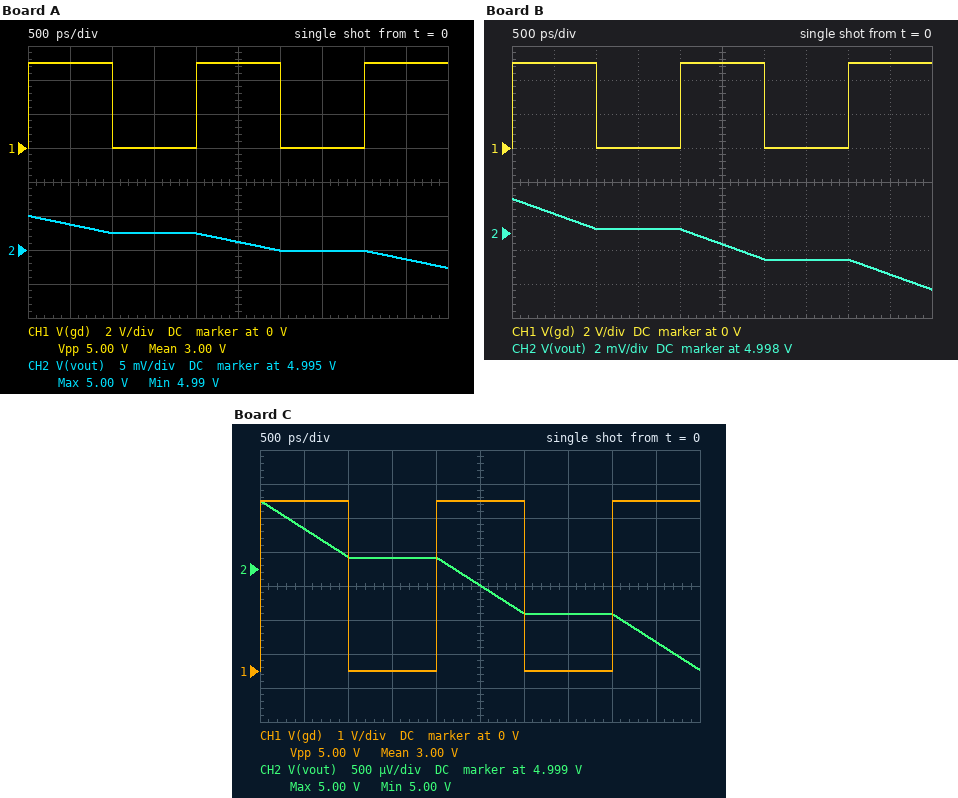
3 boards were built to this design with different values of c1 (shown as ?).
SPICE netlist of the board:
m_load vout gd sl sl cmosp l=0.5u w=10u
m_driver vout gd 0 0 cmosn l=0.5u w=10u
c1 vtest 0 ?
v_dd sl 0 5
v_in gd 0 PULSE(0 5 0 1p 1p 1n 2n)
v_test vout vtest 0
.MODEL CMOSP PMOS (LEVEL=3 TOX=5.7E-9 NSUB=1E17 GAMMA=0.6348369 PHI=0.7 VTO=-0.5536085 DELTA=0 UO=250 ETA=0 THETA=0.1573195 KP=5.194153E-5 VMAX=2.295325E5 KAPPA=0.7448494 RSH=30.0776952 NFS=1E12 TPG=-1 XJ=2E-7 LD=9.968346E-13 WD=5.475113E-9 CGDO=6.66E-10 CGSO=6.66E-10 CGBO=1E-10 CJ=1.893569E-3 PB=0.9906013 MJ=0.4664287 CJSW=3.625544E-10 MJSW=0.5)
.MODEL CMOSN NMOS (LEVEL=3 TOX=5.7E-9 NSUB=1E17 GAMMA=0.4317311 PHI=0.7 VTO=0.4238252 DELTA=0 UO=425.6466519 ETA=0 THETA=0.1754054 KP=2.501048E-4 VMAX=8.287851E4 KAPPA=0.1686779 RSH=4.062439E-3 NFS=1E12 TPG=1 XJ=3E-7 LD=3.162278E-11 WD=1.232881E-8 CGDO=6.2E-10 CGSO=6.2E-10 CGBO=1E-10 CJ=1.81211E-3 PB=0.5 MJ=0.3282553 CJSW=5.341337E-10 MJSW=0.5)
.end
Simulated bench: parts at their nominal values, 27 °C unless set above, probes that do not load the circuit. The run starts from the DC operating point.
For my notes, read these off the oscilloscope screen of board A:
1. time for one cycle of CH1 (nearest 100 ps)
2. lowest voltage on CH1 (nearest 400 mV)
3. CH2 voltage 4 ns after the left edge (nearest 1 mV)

2.0 ns
0 V
4.995 V
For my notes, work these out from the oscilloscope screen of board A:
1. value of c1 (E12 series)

3.9 nF
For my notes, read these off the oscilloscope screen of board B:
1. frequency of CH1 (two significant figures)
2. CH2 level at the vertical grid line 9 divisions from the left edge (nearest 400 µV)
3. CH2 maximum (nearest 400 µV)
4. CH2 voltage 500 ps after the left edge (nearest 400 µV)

500 MHz
4.9956 V
5.0000 V
4.9992 V
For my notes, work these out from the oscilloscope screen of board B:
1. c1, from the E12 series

5.6 nF
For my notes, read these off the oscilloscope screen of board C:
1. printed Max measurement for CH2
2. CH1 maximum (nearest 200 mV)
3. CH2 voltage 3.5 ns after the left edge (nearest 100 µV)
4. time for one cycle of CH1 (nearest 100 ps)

5.00 V
5.0 V
4.9983 V
2.0 ns
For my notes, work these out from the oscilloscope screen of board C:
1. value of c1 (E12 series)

12 nF
